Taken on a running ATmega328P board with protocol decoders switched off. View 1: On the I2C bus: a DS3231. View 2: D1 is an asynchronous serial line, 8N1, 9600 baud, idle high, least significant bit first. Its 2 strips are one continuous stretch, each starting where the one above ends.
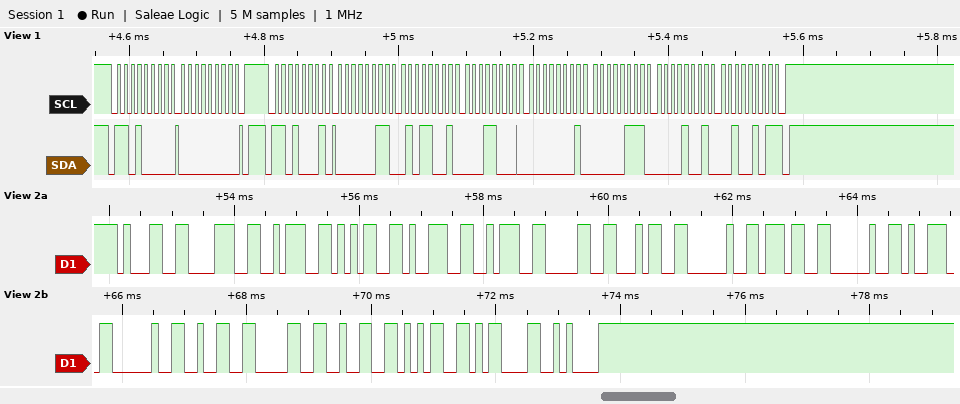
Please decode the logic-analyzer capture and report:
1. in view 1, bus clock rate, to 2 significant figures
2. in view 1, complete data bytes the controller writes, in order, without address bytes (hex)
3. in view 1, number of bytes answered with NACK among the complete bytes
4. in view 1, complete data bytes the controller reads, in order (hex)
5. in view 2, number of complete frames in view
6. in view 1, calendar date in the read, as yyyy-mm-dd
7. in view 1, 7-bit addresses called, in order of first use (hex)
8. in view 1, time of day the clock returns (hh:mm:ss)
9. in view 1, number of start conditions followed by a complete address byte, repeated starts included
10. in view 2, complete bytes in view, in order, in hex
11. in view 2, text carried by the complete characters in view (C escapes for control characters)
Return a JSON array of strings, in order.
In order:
["100 kHz", "00", "1", "03 59 18 01 07 09 25", "19", "2025-09-07", "0x68", "18:59:03", "2", "31 38 3A 35 39 3A 30 34 20 37 20 39 20 32 30 32 35 0D 0A", "\"18:59:04 7 9 2025\\r\\n\""]
